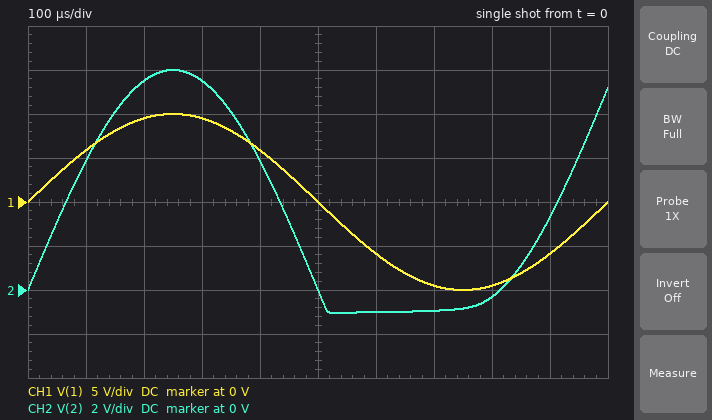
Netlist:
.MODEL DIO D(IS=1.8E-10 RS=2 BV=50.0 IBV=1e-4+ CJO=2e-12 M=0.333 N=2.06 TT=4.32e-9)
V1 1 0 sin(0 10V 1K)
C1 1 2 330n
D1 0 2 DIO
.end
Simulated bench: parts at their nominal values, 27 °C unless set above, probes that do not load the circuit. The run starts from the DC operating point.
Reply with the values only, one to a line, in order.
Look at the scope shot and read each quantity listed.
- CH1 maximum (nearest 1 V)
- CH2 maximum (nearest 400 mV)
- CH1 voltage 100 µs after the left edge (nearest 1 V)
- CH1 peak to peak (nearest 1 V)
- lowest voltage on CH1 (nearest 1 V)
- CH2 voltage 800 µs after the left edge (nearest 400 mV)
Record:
10 V
10.0 V
6 V
20 V
-10 V
-400 mV
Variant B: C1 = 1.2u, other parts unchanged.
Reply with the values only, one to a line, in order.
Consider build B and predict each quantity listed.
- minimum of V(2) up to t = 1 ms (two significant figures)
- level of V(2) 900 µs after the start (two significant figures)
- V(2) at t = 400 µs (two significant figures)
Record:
-1.2 V
3.2 V
5.9 V
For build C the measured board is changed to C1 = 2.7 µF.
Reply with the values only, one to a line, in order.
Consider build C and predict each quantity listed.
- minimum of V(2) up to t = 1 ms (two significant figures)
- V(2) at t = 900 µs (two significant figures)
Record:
-1.4 V
3.2 V
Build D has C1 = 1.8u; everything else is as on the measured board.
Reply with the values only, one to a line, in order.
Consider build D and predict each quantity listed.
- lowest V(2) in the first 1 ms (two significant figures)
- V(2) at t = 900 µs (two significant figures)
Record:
-1.3 V
3.2 V
